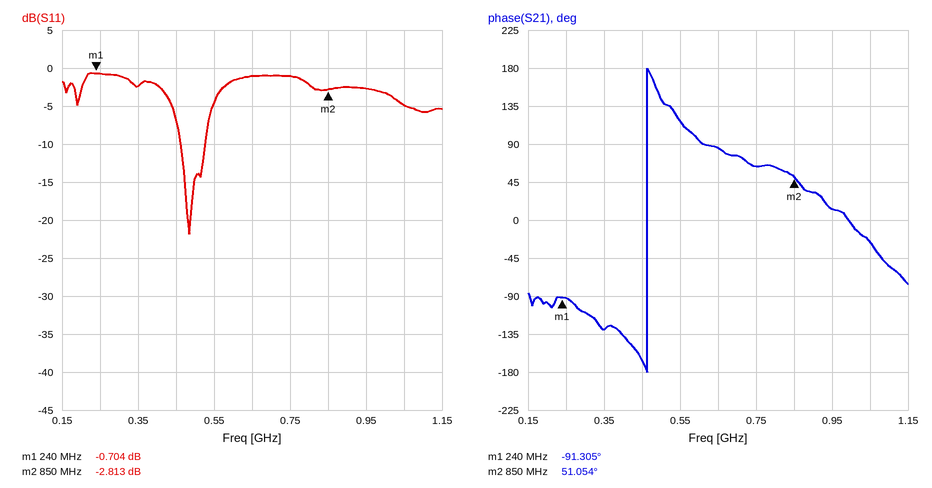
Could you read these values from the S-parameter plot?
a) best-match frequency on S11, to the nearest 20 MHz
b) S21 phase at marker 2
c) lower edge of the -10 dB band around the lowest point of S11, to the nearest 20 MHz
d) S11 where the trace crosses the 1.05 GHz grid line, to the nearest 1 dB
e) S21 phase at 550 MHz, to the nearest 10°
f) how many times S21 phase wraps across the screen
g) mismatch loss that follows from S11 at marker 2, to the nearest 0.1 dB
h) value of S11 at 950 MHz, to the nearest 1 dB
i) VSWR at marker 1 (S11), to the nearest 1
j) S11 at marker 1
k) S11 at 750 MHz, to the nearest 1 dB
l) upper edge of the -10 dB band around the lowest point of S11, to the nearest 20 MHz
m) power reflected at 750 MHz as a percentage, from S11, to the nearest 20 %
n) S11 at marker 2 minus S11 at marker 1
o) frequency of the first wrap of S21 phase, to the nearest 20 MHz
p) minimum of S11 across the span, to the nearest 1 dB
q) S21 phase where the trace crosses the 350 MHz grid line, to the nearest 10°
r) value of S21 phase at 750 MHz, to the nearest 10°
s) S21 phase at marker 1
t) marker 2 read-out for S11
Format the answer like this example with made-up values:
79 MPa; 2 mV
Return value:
480 MHz; 51.054°; 460 MHz; -5 dB; 120°; 1; 3.2 dB; -3 dB; 25; -0.704 dB; -1 dB; 520 MHz; 80 %; -2.109 dB; 460 MHz; -22 dB; -130°; 60°; -91.305°; -2.813 dB
